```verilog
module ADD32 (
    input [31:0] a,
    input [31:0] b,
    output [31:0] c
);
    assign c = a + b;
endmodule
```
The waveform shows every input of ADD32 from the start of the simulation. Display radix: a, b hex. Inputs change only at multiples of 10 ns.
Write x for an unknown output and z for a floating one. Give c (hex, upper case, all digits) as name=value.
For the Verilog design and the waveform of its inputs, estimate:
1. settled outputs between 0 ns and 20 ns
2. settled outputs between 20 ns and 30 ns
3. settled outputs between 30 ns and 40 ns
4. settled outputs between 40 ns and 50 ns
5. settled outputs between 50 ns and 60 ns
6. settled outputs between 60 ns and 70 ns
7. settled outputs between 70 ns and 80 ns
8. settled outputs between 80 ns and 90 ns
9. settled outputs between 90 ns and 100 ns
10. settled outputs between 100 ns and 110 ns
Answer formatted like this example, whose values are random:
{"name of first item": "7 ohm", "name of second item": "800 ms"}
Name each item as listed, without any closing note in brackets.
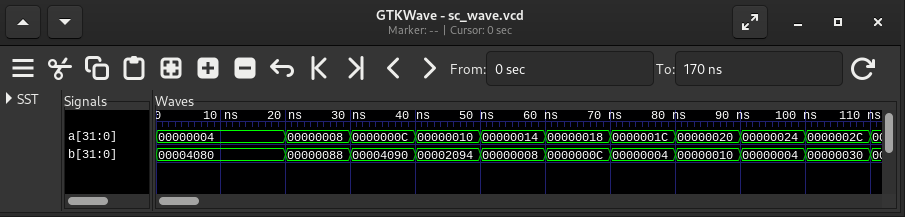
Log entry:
{"settled outputs between 0 ns and 20 ns": "c=00004084", "settled outputs between 20 ns and 30 ns": "c=00000090", "settled outputs between 30 ns and 40 ns": "c=0000409C", "settled outputs between 40 ns and 50 ns": "c=000020A4", "settled outputs between 50 ns and 60 ns": "c=0000001C", "settled outputs between 60 ns and 70 ns": "c=00000024", "settled outputs between 70 ns and 80 ns": "c=00000020", "settled outputs between 80 ns and 90 ns": "c=00000030", "settled outputs between 90 ns and 100 ns": "c=00000028", "settled outputs between 100 ns and 110 ns": "c=0000005C"}
